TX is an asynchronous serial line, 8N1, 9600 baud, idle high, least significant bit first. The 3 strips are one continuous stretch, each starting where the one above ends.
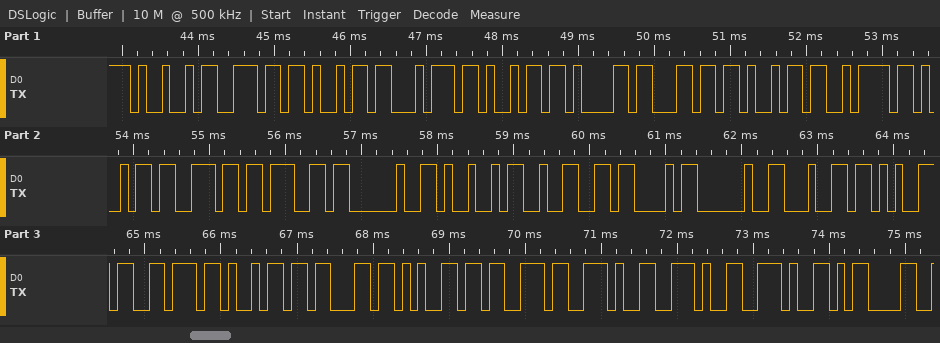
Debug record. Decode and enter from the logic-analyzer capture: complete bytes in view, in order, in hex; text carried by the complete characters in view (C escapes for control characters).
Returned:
0x49 0x6E 0x69 0x74 0x69 0x61 0x6C 0x69 0x7A 0x69 0x6E 0x67 0x20 0x49 0x32 0x43 0x20 0x64 0x65 0x76 0x69 0x63 0x65 0x73 0x2E 0x2E 0x2E 0x0D
"Initializing I2C devices...\r"
